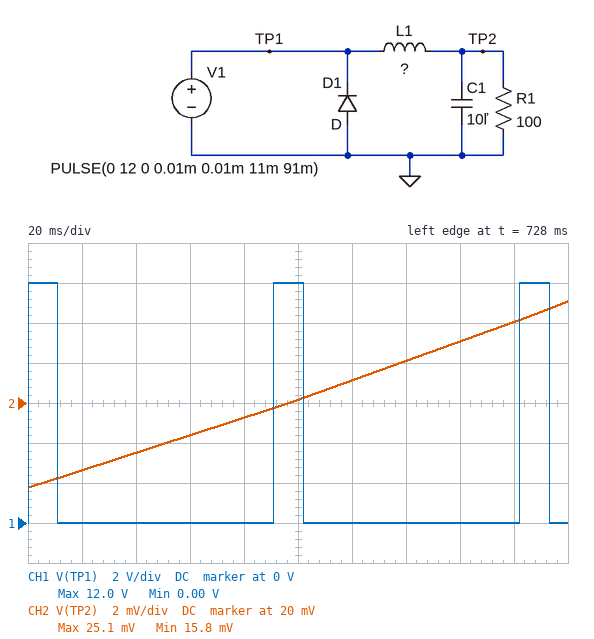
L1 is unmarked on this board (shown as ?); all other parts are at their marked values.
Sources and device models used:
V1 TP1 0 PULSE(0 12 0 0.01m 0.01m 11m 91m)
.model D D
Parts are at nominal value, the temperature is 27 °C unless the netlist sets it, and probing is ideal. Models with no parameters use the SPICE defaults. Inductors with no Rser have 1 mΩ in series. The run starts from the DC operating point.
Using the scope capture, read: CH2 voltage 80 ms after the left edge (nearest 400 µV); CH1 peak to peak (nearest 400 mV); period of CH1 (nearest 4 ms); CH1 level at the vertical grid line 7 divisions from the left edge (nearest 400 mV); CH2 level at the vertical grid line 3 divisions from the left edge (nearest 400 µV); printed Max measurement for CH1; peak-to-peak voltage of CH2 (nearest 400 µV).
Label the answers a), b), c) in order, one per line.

a) 19.2 mV
b) 12.0 V
c) 92 ms
d) 0 V
e) 18.4 mV
f) 12.0 V
g) 9.2 mV
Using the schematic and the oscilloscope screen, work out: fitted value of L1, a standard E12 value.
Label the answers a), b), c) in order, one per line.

a) 2.7 H
